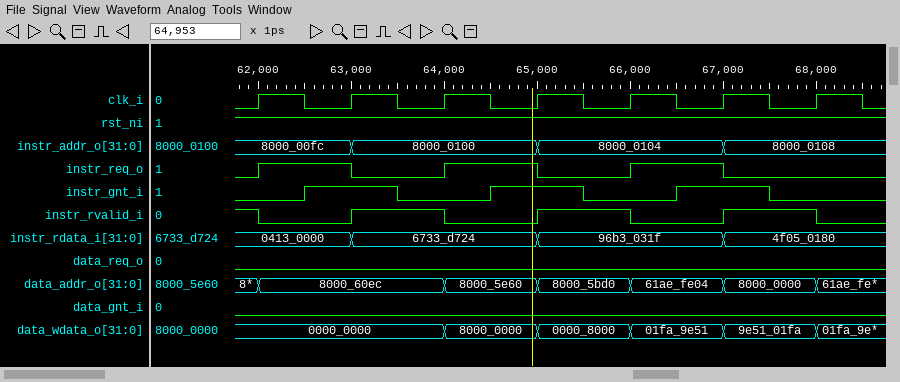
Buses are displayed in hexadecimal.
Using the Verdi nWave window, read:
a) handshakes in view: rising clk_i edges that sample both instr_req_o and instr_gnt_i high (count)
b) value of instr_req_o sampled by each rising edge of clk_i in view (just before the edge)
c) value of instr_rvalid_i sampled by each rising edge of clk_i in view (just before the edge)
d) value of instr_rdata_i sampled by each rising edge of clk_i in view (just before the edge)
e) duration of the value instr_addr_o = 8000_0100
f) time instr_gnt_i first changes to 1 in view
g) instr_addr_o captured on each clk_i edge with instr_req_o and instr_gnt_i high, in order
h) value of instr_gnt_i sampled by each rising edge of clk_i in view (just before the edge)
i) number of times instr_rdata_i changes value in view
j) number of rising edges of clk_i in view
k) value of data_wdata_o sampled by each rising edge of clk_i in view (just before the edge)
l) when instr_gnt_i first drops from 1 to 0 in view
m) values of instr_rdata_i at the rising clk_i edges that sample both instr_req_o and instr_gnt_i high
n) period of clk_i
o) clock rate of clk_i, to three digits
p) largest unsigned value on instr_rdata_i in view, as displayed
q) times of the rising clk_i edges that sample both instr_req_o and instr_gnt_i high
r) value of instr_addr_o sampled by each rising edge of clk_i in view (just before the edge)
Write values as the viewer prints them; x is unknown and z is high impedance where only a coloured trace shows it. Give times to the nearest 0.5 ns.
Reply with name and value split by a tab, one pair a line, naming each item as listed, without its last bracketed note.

handshakes in view: rising clk_i edges that sample both instr_req_o and instr_gnt_i high	3
value of instr_req_o sampled by each rising edge of clk_i in view	0 1 0 1 0 1 0
value of instr_rvalid_i sampled by each rising edge of clk_i in view	1 0 1 0 1 0 1
value of instr_rdata_i sampled by each rising edge of clk_i in view	0413_0000, 0413_0000, 6733_d724, 6733_d724, 96b3_031f, 96b3_031f, 4f05_0180
duration of the value instr_addr_o = 8000_0100	2 ns
time instr_gnt_i first changes to 1 in view	62.5 ns
instr_addr_o captured on each clk_i edge with instr_req_o and instr_gnt_i high, in order	8000_00fc, 8000_0100, 8000_0104
value of instr_gnt_i sampled by each rising edge of clk_i in view	0 1 0 1 0 1 0
number of times instr_rdata_i changes value in view	3
number of rising edges of clk_i in view	7
value of data_wdata_o sampled by each rising edge of clk_i in view	0000_0000, 0000_0000, 0000_0000, 8000_0000, 0000_8000, 01fa_9e51, 9e51_01fa
when instr_gnt_i first drops from 1 to 0 in view	63.5 ns
values of instr_rdata_i at the rising clk_i edges that sample both instr_req_o and instr_gnt_i high	0413_0000, 6733_d724, 96b3_031f
period of clk_i	1 ns
clock rate of clk_i, to three digits	1.00 GHz
largest unsigned value on instr_rdata_i in view, as displayed	96b3_031f
times of the rising clk_i edges that sample both instr_req_o and instr_gnt_i high	63 ns, 65 ns, 67 ns
value of instr_addr_o sampled by each rising edge of clk_i in view	8000_00fc, 8000_00fc, 8000_0100, 8000_0100, 8000_0104, 8000_0104, 8000_0108
